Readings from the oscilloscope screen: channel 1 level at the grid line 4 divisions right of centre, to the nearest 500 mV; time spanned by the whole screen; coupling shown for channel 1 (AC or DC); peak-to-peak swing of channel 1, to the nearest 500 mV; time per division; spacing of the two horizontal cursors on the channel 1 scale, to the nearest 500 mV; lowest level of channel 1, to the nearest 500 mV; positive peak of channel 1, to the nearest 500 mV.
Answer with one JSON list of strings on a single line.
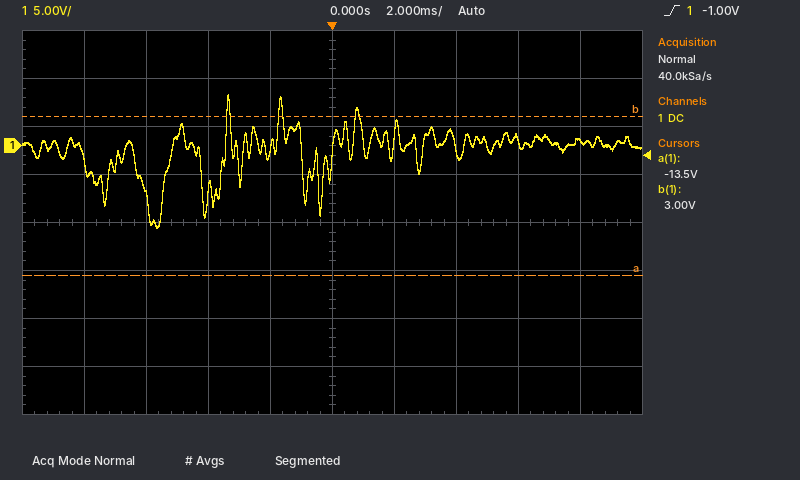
["500 mV", "20 ms", "DC", "14.0 V", "2 ms", "16.5 V", "-8.5 V", "5.5 V"]
